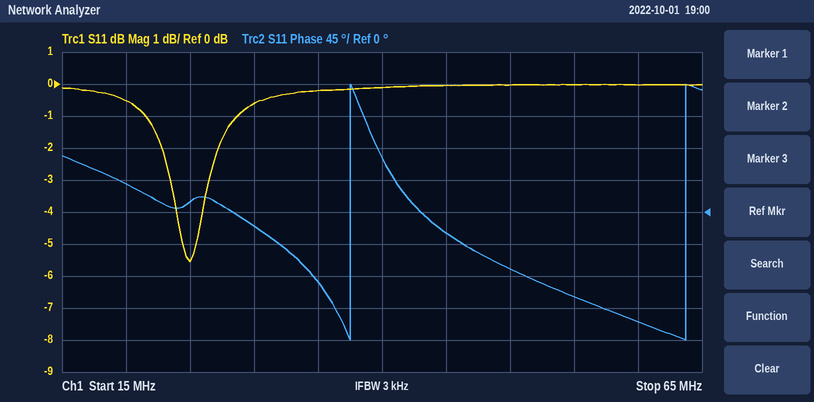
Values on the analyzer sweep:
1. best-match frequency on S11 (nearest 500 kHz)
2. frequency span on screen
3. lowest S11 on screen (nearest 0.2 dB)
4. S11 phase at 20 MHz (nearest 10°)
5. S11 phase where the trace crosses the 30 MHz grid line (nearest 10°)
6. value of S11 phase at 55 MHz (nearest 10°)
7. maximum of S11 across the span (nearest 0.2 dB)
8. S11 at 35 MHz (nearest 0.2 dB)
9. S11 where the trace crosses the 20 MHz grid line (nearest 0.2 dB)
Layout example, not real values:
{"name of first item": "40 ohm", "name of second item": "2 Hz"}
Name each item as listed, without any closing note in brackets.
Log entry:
{"best-match frequency on S11": "25.0 MHz", "frequency span on screen": "50 MHz", "lowest S11 on screen": "-5.6 dB", "S11 phase at 20 MHz": "40°", "S11 phase where the trace crosses the 30 MHz grid line": "-20°", "value of S11 phase at 55 MHz": "-120°", "maximum of S11 across the span": "0.0 dB", "S11 at 35 MHz": "-0.2 dB", "S11 where the trace crosses the 20 MHz grid line": "-0.6 dB"}
